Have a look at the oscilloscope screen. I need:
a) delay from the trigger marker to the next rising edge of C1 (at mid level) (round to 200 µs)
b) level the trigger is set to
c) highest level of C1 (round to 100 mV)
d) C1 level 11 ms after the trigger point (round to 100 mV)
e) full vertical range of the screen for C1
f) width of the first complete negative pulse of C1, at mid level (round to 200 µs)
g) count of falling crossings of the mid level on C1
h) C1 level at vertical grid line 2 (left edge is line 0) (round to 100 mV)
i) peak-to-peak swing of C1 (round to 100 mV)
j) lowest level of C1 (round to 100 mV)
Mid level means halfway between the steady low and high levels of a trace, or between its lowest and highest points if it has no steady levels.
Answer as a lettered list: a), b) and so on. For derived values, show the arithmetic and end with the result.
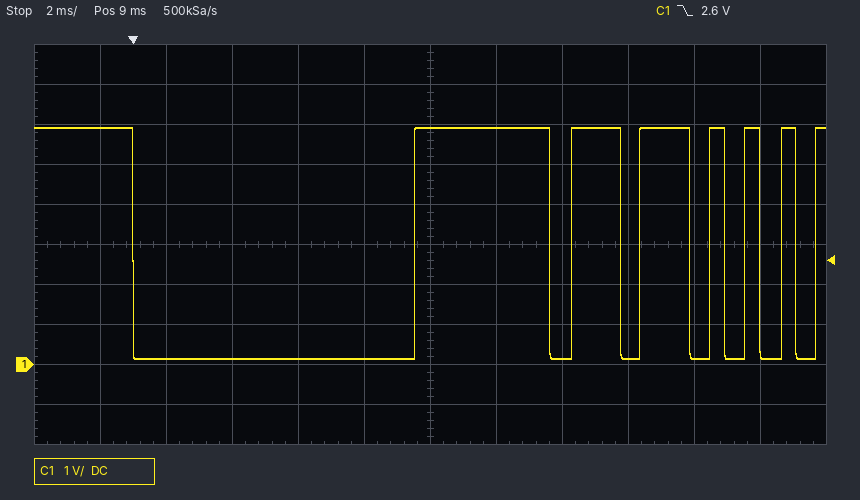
a) 8.6 ms
b) 2.6 V
c) 5.9 V
d) 5.9 V
e) 10 V
f) 8.6 ms
g) 7
h) 100 mV
i) 5.9 V − (100 mV) = 5.8 V
j) 100 mV
